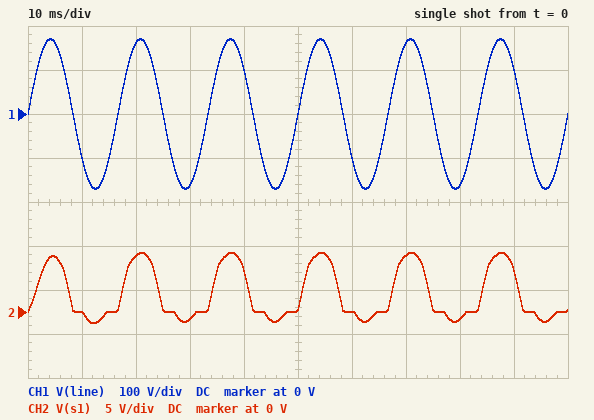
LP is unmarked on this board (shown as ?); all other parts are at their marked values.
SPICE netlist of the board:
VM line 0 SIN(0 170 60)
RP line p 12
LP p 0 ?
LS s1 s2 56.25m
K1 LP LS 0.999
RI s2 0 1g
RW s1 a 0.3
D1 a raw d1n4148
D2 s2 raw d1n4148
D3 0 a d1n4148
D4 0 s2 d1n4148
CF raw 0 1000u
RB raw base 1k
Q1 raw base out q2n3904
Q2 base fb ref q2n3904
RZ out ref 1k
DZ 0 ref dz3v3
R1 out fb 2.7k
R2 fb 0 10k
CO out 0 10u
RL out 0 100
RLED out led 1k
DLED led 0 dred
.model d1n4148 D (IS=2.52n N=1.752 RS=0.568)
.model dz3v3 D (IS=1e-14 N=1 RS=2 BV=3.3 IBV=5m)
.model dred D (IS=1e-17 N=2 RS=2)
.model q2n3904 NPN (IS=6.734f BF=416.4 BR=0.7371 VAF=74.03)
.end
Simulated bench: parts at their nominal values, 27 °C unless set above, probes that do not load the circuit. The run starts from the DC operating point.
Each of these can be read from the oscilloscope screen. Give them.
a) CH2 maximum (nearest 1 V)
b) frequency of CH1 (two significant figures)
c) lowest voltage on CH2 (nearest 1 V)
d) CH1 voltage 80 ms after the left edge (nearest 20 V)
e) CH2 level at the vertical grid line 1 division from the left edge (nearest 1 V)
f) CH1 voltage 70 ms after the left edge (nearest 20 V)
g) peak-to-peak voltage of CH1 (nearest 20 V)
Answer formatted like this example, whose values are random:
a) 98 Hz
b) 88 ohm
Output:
a) 7 V
b) 60 Hz
c) -1 V
d) -160 V
e) 0 V
f) 160 V
g) 340 V
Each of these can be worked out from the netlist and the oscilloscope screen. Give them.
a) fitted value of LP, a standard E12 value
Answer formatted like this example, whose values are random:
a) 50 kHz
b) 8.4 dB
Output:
a) 27 H
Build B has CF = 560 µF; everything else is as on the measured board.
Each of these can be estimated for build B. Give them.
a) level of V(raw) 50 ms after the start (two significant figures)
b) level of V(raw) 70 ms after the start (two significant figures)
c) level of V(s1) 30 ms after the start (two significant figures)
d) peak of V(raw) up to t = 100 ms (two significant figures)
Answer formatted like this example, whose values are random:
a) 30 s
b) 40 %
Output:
a) 5.6 V
b) 5.4 V
c) -780 mV
d) 5.9 V
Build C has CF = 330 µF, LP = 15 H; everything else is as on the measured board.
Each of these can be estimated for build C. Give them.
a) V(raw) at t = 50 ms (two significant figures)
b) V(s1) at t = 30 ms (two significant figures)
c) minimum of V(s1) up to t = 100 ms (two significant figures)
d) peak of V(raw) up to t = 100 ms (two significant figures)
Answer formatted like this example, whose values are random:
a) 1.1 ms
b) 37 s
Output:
a) 8.0 V
b) -680 mV
c) -1.2 V
d) 8.6 V
